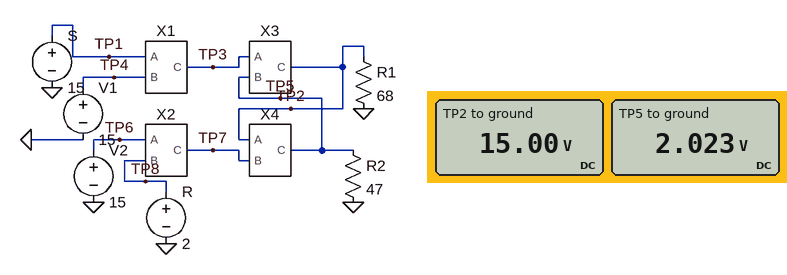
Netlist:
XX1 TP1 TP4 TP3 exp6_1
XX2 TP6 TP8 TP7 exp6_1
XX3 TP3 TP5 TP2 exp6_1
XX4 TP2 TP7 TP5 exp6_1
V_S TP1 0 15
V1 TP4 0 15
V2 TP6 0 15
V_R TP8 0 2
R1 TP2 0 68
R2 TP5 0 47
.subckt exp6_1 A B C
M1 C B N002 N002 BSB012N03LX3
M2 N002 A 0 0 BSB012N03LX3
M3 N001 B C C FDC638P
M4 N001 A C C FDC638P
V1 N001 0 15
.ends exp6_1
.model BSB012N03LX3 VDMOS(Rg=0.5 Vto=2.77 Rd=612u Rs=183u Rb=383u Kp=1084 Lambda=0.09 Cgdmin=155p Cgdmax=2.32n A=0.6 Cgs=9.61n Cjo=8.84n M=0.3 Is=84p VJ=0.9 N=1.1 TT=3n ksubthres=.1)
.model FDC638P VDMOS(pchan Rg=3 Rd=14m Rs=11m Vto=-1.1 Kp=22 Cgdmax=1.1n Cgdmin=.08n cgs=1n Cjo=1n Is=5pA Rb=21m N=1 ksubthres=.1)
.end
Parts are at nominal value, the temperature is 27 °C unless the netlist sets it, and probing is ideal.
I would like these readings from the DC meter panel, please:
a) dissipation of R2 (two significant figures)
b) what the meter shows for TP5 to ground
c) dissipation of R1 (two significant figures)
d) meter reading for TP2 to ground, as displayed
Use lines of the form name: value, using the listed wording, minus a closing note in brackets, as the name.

dissipation of R2: 87 mW
what the meter shows for TP5 to ground: 2.023 V
dissipation of R1: 3.3 W
meter reading for TP2 to ground, as displayed: 15.00 V
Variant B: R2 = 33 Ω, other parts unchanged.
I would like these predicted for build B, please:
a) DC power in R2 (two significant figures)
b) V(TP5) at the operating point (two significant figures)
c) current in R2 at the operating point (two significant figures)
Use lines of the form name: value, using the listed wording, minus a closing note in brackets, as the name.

DC power in R2: 120 mW
V(TP5) at the operating point: 2.0 V
current in R2 at the operating point: 61 mA
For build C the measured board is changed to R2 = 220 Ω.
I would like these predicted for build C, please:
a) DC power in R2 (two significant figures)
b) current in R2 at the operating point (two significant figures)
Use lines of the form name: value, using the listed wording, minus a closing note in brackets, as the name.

DC power in R2: 19 mW
current in R2 at the operating point: 9.2 mA
